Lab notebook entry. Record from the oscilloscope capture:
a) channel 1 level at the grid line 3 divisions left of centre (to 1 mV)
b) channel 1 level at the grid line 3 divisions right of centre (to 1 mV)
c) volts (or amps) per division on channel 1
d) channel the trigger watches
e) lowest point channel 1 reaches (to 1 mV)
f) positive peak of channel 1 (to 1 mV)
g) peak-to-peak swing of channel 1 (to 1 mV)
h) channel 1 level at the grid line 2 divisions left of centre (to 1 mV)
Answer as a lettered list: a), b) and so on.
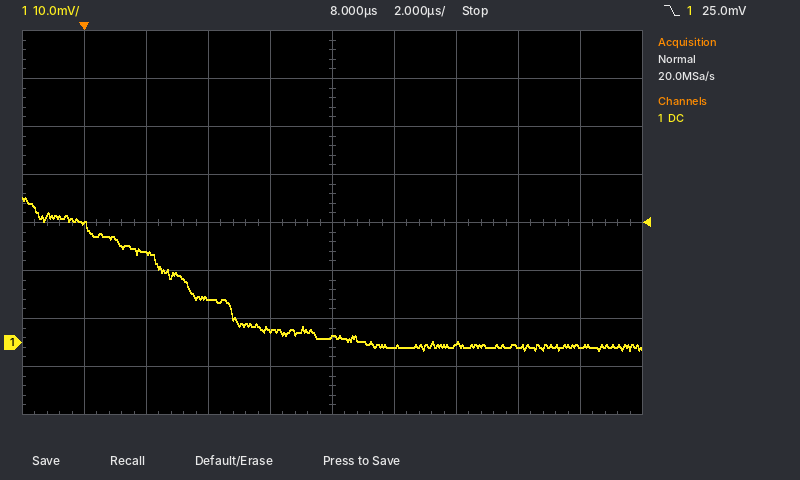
a) 19 mV
b) -1 mV
c) 10 mV
d) channel 1
e) -2 mV
f) 30 mV
g) 32 mV
h) 9 mV
